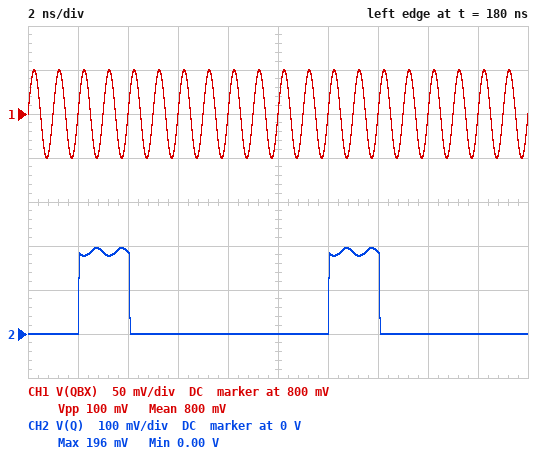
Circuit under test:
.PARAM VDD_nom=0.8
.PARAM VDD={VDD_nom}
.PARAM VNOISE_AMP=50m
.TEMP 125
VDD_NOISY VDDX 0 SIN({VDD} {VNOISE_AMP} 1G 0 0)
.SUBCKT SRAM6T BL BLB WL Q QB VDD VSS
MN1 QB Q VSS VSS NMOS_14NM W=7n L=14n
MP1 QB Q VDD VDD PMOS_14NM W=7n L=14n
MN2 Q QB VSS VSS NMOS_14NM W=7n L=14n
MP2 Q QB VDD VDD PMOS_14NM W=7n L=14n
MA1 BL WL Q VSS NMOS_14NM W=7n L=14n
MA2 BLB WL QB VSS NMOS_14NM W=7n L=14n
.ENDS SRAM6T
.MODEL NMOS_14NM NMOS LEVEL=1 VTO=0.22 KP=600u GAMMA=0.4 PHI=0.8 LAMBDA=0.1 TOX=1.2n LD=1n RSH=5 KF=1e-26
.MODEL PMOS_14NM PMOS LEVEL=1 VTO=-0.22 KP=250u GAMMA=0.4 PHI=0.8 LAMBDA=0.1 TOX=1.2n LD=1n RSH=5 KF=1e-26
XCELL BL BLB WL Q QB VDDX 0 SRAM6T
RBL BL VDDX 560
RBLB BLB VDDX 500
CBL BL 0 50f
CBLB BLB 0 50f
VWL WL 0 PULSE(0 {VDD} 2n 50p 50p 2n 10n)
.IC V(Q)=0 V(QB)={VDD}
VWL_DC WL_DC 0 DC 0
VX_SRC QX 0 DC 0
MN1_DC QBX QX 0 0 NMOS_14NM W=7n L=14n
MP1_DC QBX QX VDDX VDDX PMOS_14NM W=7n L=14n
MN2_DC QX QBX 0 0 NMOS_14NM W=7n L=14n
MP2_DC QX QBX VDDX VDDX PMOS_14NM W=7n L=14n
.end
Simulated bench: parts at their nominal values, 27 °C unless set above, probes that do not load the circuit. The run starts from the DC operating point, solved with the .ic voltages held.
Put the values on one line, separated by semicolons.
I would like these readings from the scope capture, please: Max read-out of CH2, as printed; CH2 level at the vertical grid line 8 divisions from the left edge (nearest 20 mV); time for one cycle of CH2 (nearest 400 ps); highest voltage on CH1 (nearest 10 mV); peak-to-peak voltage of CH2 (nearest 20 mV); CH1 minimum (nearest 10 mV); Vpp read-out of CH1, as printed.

196 mV; 0 V; 10.0 ns; 850 mV; 200 mV; 750 mV; 100 mV
